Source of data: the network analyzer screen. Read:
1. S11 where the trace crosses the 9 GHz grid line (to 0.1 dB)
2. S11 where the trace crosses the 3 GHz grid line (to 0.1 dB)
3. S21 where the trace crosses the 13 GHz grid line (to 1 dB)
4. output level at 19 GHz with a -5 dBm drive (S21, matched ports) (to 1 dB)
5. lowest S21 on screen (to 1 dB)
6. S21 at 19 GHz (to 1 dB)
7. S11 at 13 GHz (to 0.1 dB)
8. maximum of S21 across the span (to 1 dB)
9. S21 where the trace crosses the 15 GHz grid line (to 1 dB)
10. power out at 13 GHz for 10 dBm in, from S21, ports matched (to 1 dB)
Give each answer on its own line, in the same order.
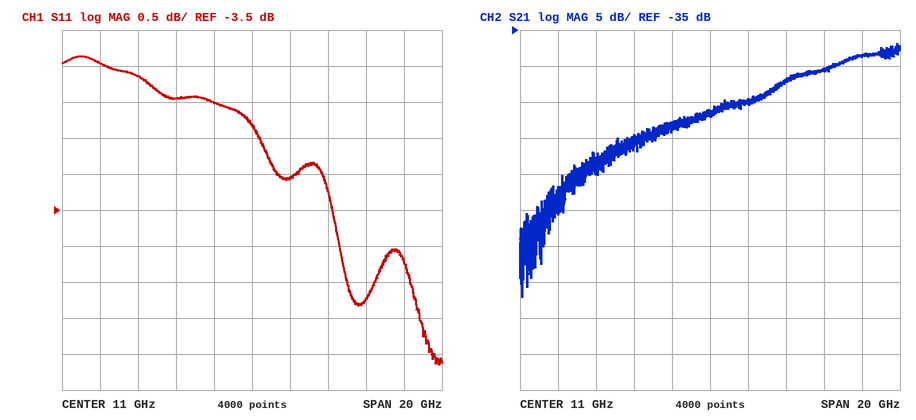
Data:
-2.0 dB
-1.5 dB
-45 dB
-44 dBm
-72 dB
-39 dB
-3.1 dB
-37 dB
-42 dB
-35 dBm
